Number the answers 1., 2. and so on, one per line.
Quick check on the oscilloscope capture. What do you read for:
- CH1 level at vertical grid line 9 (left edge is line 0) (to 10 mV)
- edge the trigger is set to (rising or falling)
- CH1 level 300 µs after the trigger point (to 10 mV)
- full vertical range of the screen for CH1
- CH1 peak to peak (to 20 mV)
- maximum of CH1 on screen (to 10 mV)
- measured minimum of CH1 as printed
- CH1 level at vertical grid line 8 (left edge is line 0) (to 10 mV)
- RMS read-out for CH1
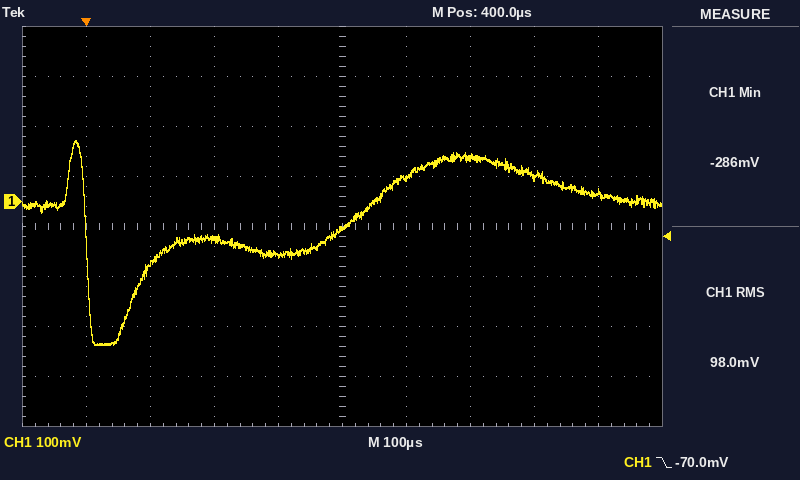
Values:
1. 20 mV
2. falling
3. -110 mV
4. 800 mV
5. 400 mV
6. 120 mV
7. -286 mV
8. 50 mV
9. 98.0 mV
